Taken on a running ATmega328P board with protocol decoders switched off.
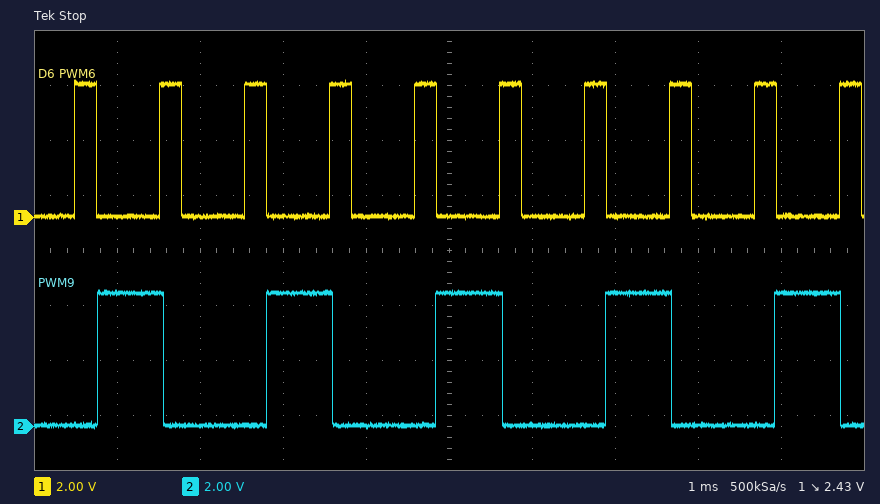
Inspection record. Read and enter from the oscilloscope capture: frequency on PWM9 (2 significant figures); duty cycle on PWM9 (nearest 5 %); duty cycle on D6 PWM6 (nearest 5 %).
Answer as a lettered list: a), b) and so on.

a) 490 Hz
b) 40 %
c) 25 %
